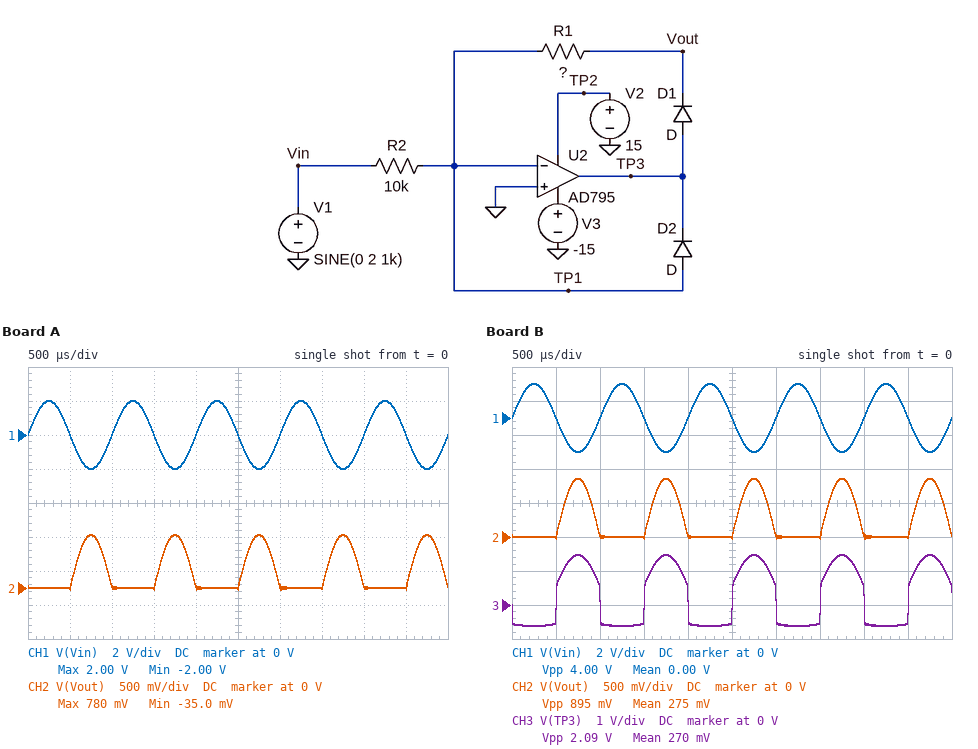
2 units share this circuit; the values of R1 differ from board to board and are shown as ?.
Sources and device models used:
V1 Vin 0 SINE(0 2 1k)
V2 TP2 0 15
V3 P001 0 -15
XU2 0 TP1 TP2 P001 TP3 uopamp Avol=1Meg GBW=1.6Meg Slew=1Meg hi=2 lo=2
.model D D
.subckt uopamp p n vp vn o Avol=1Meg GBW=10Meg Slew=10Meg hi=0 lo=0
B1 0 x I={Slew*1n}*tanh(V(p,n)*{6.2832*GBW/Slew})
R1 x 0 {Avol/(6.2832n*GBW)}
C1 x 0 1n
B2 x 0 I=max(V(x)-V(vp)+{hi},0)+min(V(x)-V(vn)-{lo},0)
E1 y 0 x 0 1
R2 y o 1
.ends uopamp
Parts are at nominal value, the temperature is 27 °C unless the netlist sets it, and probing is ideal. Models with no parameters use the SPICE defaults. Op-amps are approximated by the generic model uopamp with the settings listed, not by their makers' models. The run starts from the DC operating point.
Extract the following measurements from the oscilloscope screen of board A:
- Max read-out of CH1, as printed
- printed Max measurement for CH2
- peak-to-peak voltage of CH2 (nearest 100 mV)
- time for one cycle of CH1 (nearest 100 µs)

2.00 V
780 mV
800 mV
1.0 ms
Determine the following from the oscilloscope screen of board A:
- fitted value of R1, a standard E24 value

3.9 kΩ
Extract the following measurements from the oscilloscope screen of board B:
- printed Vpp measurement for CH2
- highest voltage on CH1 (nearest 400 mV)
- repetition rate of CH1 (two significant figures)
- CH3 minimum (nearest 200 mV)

895 mV
2.0 V
1.0 kHz
-600 mV
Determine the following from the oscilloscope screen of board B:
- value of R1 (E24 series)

4.3 kΩ
